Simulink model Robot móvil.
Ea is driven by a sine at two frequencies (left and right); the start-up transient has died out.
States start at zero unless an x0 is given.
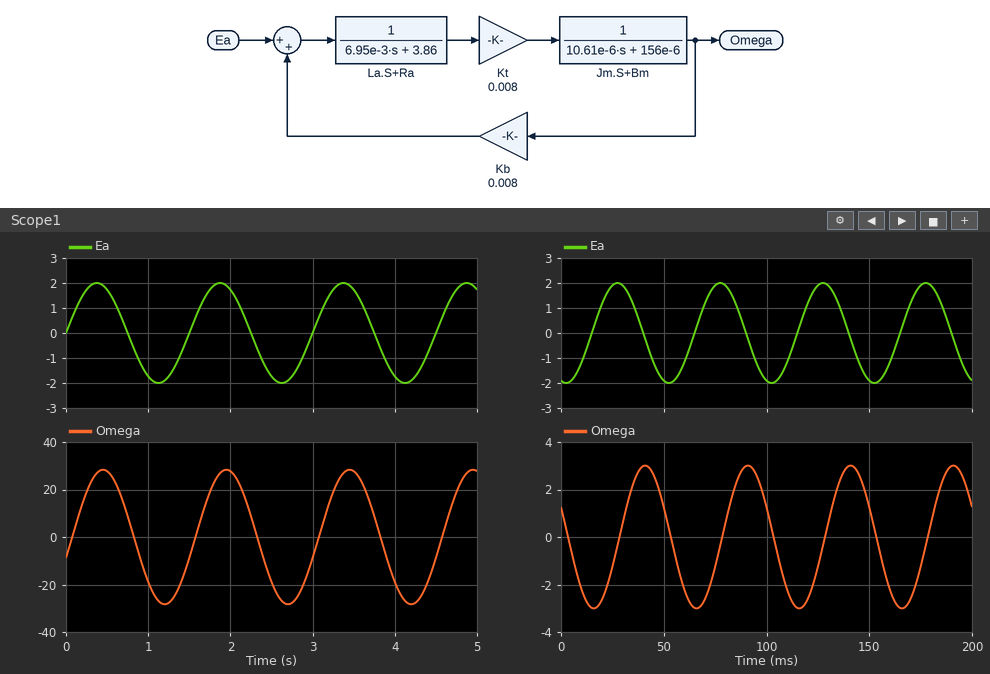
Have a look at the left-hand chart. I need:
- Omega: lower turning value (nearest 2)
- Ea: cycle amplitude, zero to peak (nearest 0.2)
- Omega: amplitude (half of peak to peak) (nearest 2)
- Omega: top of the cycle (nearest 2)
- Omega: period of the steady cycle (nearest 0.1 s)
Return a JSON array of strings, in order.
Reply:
["-28", "2.0", "28", "28", "1.5 s"]
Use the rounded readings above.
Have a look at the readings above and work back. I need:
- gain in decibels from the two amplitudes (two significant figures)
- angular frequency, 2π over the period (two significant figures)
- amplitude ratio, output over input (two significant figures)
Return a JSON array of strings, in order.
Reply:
["23 dB", "4.2 rad/s", "14"]
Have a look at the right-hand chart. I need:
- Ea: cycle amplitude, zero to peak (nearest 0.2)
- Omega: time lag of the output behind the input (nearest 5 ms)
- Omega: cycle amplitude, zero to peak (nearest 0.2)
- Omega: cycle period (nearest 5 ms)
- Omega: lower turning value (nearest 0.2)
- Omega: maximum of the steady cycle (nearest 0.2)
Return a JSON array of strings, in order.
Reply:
["2.0", "15 ms", "3.0", "50 ms", "-3.0", "3.0"]
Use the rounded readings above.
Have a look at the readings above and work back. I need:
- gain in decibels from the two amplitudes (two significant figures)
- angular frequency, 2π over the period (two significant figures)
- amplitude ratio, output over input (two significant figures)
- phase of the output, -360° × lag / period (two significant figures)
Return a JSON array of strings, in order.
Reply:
["3.5 dB", "0.13 rad/ms", "1.5", "-110°"]
